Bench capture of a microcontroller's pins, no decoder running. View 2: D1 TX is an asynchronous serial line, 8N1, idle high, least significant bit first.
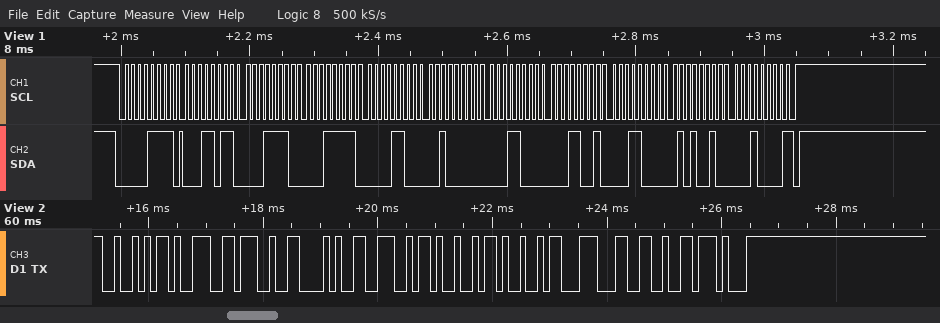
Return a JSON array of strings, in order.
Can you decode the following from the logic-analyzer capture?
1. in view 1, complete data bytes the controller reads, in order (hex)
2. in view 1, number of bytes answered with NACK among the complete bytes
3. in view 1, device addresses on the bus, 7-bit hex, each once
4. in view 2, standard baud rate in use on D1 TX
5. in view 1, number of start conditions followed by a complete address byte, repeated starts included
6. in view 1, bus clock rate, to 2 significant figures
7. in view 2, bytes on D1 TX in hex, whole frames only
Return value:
["1B 1E 1F 0C 20 18 19 18 52 10", "1", "0x07", "9600 baud", "1", "100 kHz", "52 39 27 28 4E 49 49 1C 26 17"]
